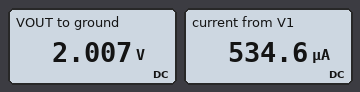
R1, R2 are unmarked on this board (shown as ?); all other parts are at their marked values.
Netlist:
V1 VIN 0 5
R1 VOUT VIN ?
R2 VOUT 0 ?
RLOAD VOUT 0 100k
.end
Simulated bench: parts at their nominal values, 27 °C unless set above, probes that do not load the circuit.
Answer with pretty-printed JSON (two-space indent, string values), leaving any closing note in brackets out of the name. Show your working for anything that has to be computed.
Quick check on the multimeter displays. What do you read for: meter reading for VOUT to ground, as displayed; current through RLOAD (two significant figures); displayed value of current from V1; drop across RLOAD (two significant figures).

{
  "meter reading for VOUT to ground, as displayed": "2.007 V",
  "current through RLOAD": "(2.007 V) / 100 kΩ = 20 µA",
  "displayed value of current from V1": "534.6 µA",
  "drop across RLOAD": "2.007 V = 2.0 V"
}
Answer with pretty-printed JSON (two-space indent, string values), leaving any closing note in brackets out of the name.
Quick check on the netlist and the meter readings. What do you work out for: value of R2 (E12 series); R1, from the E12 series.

{
  "value of R2": "3.9 kΩ",
  "R1, from the E12 series": "5.6 kΩ"
}
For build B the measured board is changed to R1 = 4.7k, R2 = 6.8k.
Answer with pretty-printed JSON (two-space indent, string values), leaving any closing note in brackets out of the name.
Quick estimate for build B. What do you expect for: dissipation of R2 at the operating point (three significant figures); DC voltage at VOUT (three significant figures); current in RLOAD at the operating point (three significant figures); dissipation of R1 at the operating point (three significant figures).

{
  "dissipation of R2 at the operating point": "1.22 mW",
  "DC voltage at VOUT": "2.88 V",
  "current in RLOAD at the operating point": "28.8 µA",
  "dissipation of R1 at the operating point": "959 µW"
}
